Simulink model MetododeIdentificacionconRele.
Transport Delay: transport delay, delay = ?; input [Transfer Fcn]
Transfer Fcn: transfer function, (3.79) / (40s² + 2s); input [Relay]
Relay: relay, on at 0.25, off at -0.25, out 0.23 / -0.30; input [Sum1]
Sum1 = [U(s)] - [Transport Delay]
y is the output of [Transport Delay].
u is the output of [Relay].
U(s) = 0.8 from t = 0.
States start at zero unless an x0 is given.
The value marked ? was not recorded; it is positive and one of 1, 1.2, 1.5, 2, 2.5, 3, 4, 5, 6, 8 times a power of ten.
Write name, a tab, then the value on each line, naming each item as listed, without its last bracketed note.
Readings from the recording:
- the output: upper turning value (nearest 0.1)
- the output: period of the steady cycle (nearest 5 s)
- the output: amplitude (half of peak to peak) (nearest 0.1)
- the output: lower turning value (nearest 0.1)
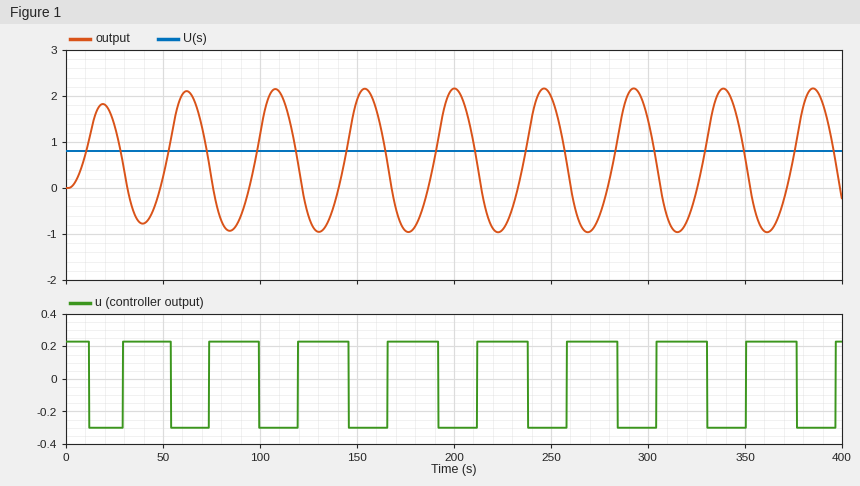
the output: upper turning value	2.2
the output: period of the steady cycle	45 s
the output: amplitude (half of peak to peak)	1.6
the output: lower turning value	-1.0
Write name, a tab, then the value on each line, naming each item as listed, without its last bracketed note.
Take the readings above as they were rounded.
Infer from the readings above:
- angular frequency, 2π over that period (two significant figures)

angular frequency, 2π over that period	0.14 rad/s
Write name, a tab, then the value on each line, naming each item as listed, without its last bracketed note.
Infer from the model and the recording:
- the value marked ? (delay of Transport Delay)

the value marked ?	1.2
